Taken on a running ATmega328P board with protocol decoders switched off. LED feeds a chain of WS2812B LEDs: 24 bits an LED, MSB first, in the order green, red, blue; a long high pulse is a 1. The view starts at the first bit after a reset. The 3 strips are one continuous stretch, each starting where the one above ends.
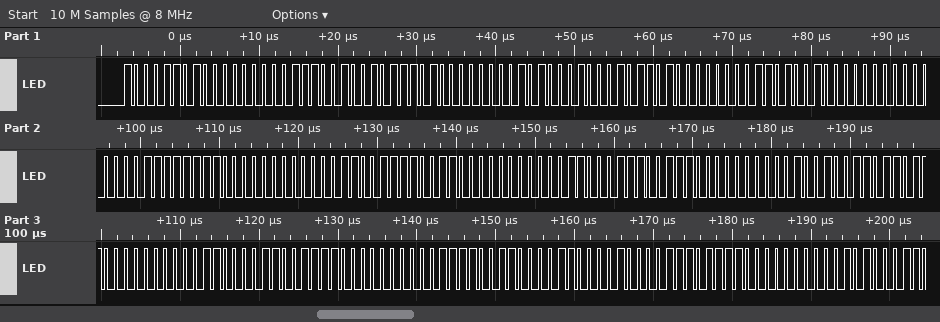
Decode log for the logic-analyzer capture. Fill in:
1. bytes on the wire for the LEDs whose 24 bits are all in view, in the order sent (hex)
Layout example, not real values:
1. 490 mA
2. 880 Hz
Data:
1. 8D 00 72 5D 00 A2 2D 00 D2 00 03 FC 00 33 CC 00 63 9C 00 93 6C 00 C3 3C 00 F3 0C 21 DE 00
